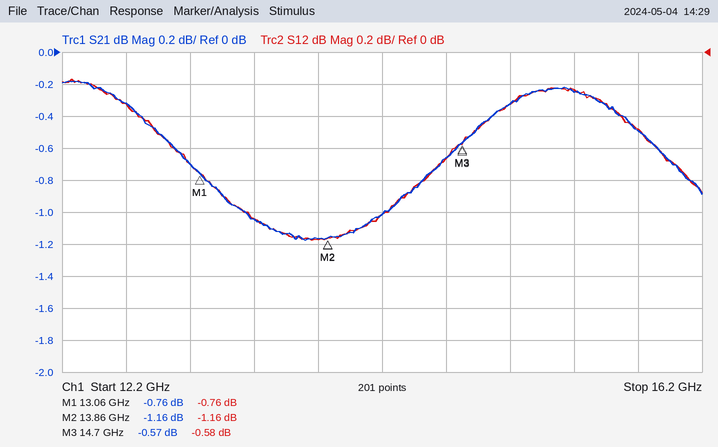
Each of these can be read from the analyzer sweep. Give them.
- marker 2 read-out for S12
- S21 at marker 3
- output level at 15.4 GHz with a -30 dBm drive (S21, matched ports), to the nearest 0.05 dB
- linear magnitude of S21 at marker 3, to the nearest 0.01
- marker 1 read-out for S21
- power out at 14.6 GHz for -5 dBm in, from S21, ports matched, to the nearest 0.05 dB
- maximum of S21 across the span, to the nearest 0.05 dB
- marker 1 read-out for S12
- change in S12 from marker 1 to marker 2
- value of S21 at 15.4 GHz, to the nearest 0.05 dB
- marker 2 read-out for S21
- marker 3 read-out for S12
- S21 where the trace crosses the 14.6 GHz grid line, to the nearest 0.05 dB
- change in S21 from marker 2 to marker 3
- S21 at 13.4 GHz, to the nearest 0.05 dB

-1.16 dB
-0.57 dB
-30.25 dBm
0.94
-0.76 dB
-5.65 dBm
-0.20 dB
-0.76 dB
-0.40 dB
-0.25 dB
-1.16 dB
-0.58 dB
-0.65 dB
0.59 dB
-1.05 dB
